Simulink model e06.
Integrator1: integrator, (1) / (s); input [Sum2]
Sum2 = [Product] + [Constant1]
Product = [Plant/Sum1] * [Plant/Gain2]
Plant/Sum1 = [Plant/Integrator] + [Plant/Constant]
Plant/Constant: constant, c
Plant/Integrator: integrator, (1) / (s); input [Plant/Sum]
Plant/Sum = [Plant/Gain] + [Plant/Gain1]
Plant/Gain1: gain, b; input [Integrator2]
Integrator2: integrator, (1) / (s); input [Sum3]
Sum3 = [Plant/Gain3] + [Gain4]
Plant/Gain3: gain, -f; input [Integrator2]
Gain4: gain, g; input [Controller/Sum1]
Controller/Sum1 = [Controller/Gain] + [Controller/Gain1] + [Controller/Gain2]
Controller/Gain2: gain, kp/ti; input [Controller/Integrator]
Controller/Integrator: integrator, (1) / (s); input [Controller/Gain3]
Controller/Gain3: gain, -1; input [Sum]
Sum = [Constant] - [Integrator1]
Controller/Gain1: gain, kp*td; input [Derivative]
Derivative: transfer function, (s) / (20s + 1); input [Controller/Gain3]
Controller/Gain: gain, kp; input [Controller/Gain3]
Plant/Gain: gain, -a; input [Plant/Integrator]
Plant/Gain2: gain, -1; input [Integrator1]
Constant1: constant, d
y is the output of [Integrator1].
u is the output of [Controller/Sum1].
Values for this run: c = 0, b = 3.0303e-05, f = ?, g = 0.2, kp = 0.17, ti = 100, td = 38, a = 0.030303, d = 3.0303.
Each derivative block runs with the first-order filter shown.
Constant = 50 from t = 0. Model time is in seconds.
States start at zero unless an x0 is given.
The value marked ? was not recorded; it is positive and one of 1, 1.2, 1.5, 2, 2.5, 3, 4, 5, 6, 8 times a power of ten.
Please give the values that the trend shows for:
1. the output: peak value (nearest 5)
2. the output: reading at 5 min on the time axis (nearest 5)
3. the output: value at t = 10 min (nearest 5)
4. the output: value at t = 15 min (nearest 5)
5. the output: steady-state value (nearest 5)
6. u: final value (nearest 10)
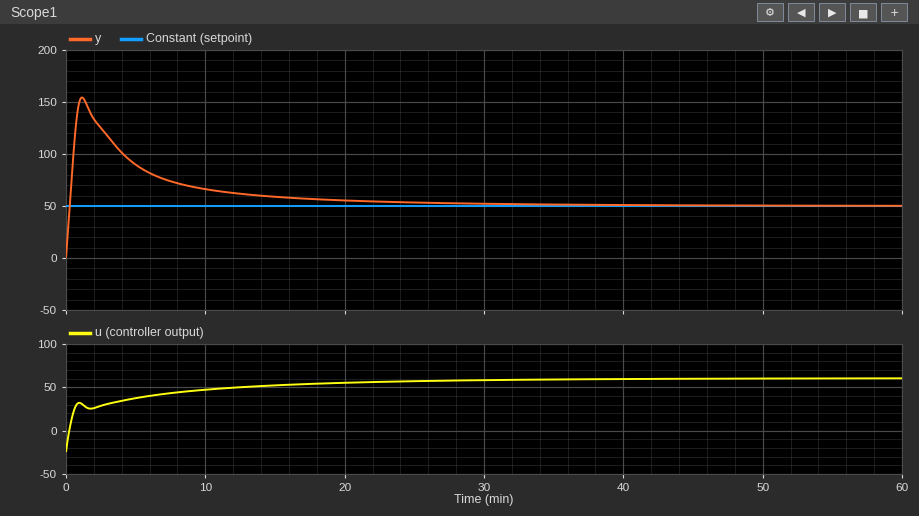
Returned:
155
90
65
60
50
60
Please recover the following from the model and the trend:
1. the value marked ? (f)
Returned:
0.2
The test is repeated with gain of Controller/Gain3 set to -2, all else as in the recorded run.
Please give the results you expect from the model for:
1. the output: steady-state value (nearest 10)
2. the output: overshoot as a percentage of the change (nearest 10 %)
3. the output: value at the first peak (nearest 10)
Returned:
50
160 %
130
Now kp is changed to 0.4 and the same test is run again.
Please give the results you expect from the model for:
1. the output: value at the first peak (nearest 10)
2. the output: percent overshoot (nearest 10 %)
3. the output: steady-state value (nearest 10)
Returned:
130
150 %
50
